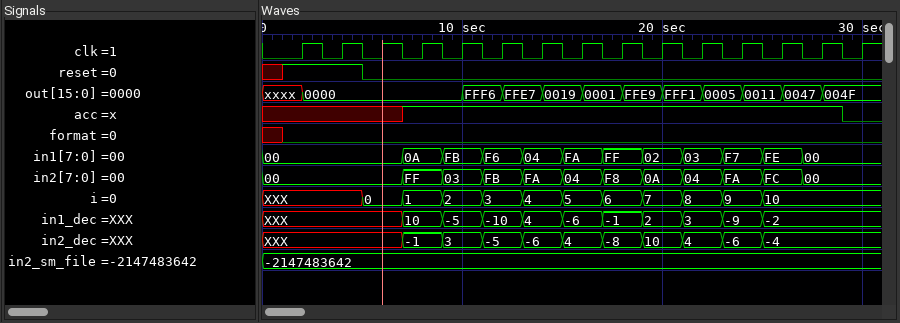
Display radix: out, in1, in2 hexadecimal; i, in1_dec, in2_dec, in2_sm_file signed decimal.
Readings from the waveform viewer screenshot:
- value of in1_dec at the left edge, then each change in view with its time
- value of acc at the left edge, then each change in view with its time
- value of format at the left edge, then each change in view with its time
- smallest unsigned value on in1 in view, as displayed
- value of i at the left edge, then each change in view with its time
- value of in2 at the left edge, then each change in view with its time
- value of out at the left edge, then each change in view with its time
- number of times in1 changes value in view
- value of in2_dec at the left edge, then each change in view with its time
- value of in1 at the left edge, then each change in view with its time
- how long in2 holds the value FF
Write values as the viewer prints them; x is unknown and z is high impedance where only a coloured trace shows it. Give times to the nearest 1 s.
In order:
XXX, 10 at 7 s, -5 at 9 s, -10 at 11 s, 4 at 13 s, -6 at 15 s, -1 at 17 s, 2 at 19 s, 3 at 21 s, -9 at 23 s, -2 at 25 s
x, 1 at 7 s, 0 at 29 s
x, 0 at 1 s
00
XXX, 0 at 5 s, 1 at 7 s, 2 at 9 s, 3 at 11 s, 4 at 13 s, 5 at 15 s, 6 at 17 s, 7 at 19 s, 8 at 21 s, 9 at 23 s, 10 at 25 s
00, FF at 7 s, 03 at 9 s, FB at 11 s, FA at 13 s, 04 at 15 s, F8 at 17 s, 0A at 19 s, 04 at 21 s, FA at 23 s, FC at 25 s, 00 at 27 s
xxxx, 0000 at 2 s, FFF6 at 10 s, FFE7 at 12 s, 0019 at 14 s, 0001 at 16 s, FFE9 at 18 s, FFF1 at 20 s, 0005 at 22 s, 0011 at 24 s, 0047 at 26 s, 004F at 28 s
11
XXX, -1 at 7 s, 3 at 9 s, -5 at 11 s, -6 at 13 s, 4 at 15 s, -8 at 17 s, 10 at 19 s, 4 at 21 s, -6 at 23 s, -4 at 25 s
00, 0A at 7 s, FB at 9 s, F6 at 11 s, 04 at 13 s, FA at 15 s, FF at 17 s, 02 at 19 s, 03 at 21 s, F7 at 23 s, FE at 25 s, 00 at 27 s
2 s
